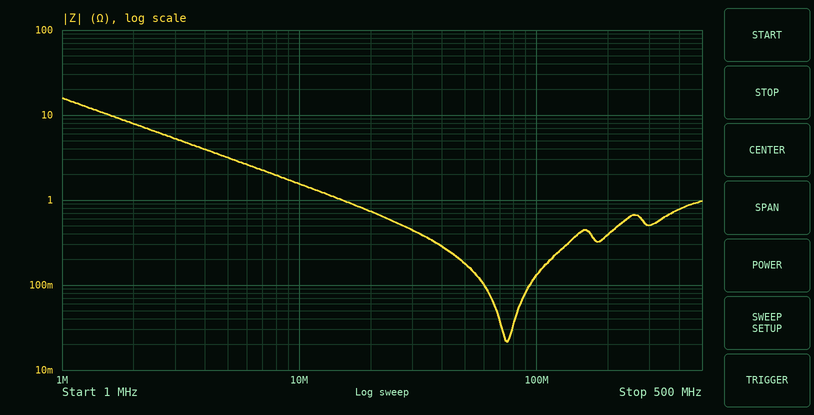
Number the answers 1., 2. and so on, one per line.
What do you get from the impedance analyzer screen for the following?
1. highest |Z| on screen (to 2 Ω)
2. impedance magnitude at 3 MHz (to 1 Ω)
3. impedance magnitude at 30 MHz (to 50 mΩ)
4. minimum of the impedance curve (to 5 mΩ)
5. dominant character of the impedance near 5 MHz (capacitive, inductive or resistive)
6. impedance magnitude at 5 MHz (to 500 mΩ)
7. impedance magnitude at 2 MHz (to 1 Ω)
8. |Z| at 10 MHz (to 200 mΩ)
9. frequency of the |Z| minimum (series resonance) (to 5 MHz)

1. 16 Ω
2. 5 Ω
3. 450 mΩ
4. 20 mΩ
5. capacitive
6. 3.0 Ω
7. 8 Ω
8. 1.6 Ω
9. 75 MHz
